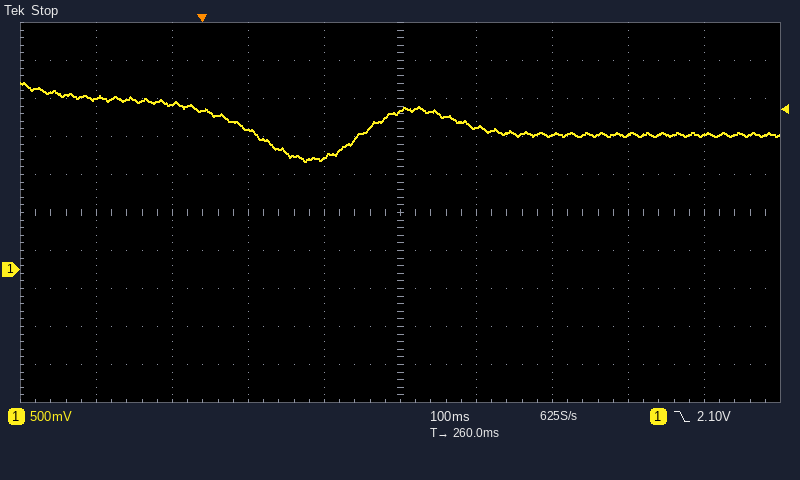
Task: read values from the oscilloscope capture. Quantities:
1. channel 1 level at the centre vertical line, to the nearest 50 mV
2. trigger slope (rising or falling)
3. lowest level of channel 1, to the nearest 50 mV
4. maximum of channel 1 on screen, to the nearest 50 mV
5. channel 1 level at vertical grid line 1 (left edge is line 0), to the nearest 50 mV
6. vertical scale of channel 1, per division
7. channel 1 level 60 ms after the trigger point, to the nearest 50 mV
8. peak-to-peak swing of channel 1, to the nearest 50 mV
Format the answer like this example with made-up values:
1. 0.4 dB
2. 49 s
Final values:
1. 2.10 V
2. falling
3. 1.40 V
4. 2.45 V
5. 2.25 V
6. 500 mV
7. 1.85 V
8. 1.05 V
